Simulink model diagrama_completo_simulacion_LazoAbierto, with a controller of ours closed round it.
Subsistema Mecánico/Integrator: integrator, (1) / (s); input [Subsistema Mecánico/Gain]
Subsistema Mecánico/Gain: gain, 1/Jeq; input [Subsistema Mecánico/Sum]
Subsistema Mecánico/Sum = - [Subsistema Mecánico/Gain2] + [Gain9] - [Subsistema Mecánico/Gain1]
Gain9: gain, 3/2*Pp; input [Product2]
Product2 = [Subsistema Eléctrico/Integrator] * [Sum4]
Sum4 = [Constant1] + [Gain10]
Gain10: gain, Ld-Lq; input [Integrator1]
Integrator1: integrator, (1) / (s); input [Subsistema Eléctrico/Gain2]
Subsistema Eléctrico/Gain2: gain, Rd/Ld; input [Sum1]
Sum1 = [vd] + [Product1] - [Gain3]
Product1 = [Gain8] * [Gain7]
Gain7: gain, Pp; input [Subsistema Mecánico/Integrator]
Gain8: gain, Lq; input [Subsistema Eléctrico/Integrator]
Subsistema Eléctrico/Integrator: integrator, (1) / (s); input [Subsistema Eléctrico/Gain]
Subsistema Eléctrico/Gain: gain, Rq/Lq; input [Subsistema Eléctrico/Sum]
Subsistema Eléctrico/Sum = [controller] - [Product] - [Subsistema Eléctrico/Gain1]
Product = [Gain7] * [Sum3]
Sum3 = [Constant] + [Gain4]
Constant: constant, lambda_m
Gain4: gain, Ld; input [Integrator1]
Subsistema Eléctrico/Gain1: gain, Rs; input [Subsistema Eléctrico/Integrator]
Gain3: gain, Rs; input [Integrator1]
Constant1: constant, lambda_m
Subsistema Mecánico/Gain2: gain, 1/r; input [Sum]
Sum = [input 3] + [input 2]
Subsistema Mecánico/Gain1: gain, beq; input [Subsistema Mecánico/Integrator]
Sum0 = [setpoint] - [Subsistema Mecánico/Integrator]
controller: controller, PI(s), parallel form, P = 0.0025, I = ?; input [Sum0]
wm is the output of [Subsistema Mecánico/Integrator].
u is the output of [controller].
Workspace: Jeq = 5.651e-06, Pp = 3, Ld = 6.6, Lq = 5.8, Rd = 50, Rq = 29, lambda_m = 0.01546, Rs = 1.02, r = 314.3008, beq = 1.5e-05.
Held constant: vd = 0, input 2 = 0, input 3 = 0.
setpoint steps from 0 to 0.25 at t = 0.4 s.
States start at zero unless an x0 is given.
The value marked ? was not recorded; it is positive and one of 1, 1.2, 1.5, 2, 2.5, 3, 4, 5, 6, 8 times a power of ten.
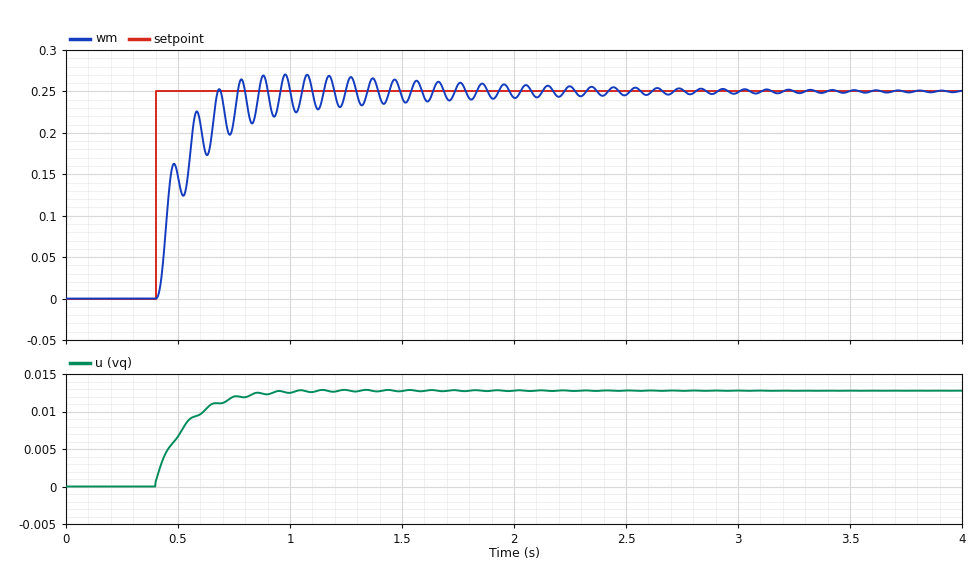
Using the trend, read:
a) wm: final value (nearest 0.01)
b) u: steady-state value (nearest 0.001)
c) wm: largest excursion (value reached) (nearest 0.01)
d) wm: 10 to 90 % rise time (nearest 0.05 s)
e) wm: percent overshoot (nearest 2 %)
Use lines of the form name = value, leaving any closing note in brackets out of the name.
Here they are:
wm: final value = 0.25
u: steady-state value = 0.013
wm: largest excursion (value reached) = 0.27
wm: 10 to 90 % rise time = 0.15 s
wm: percent overshoot = 8 %
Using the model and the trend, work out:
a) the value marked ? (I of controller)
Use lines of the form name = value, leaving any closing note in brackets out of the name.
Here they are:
the value marked ? = 0.4
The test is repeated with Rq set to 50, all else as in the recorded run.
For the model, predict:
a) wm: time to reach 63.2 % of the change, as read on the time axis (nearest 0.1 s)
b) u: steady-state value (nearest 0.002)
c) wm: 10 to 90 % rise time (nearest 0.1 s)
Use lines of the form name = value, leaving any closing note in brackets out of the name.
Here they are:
wm: time to reach 63.2 % of the change, as read on the time axis = 0.5 s
u: steady-state value = 0.012
wm: 10 to 90 % rise time = 0.3 s
